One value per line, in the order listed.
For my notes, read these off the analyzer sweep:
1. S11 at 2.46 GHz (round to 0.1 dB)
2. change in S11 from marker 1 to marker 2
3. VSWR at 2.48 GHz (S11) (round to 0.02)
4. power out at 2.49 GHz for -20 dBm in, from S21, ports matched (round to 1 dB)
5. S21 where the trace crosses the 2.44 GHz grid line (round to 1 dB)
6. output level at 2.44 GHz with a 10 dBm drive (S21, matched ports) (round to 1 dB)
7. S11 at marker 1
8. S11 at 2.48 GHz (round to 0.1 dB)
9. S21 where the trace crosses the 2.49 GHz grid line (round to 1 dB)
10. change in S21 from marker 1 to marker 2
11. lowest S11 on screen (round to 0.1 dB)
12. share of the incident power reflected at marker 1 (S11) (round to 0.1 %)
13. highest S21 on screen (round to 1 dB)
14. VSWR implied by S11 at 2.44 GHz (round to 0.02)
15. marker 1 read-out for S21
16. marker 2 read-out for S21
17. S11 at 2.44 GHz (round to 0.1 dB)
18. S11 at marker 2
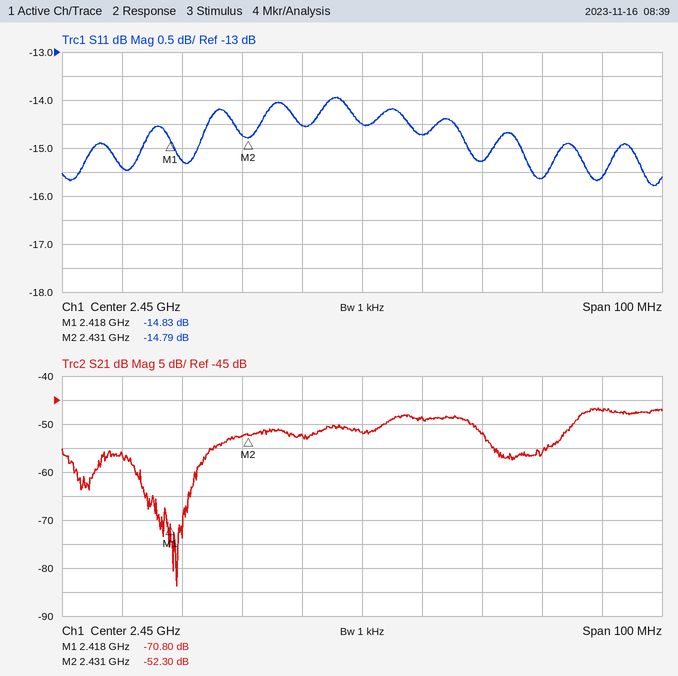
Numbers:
-14.7 dB
0.04 dB
1.40
-67 dBm
-52 dB
-42 dBm
-14.83 dB
-15.6 dB
-47 dB
18.50 dB
-15.8 dB
3.3 %
-47 dB
1.46
-70.80 dB
-52.30 dB
-14.5 dB
-14.79 dB
